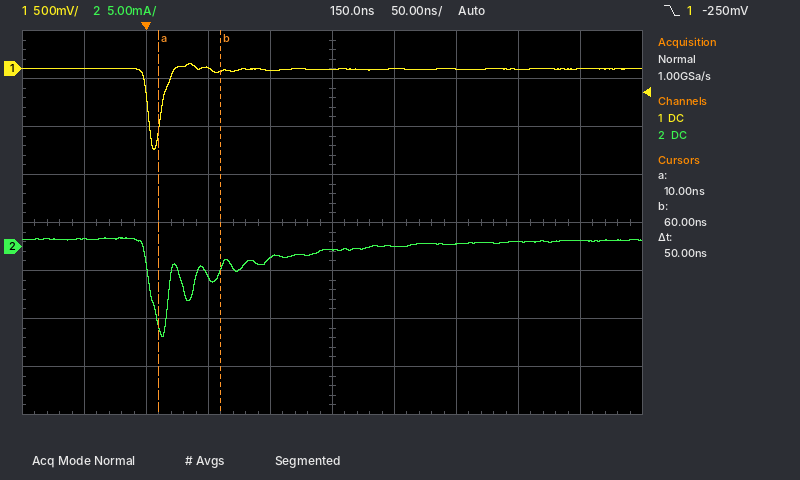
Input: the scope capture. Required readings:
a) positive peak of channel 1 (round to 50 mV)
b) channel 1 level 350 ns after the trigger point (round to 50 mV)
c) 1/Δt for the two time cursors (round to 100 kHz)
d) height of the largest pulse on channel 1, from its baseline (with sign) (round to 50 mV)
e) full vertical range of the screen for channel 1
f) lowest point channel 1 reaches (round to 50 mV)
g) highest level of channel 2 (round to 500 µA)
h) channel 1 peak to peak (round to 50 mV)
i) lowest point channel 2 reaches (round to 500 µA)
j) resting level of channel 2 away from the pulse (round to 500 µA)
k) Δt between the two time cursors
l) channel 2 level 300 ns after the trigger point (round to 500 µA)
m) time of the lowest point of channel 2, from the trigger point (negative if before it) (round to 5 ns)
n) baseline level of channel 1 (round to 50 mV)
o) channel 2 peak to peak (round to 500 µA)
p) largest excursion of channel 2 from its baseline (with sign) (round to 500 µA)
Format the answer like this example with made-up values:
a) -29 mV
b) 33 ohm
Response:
a) 50 mV
b) 0 mV
c) 20.0 MHz
d) -850 mV
e) 4 V
f) -850 mV
g) 1.0 mA
h) 900 mV
i) -9.5 mA
j) 500 µA
k) 50 ns
l) 500 µA
m) +15 ns
n) 0 mV
o) 10.5 mA
p) -10.0 mA
